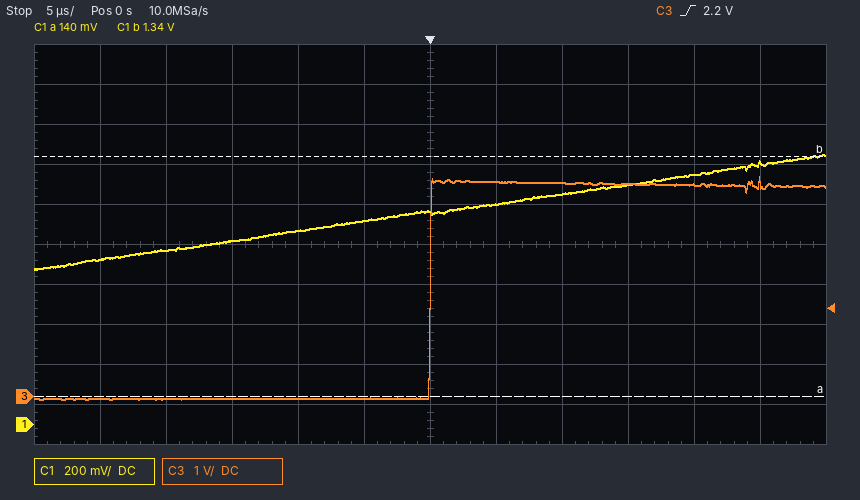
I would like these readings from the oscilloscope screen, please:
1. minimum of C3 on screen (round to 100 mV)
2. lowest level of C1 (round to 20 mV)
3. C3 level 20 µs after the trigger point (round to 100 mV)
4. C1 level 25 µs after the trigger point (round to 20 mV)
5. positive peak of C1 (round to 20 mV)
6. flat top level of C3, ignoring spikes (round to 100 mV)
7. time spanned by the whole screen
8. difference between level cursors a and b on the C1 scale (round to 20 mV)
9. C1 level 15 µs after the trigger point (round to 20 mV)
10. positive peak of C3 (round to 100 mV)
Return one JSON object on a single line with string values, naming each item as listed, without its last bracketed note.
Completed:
{"minimum of C3 on screen": "-100 mV", "lowest level of C1": "780 mV", "C3 level 20 µs after the trigger point": "5.3 V", "C1 level 25 µs after the trigger point": "1.30 V", "positive peak of C1": "1.34 V", "flat top level of C3, ignoring spikes": "5.3 V", "time spanned by the whole screen": "60 µs", "difference between level cursors a and b on the C1 scale": "1.20 V", "C1 level 15 µs after the trigger point": "1.20 V", "positive peak of C3": "5.5 V"}
